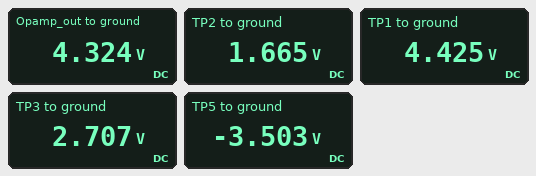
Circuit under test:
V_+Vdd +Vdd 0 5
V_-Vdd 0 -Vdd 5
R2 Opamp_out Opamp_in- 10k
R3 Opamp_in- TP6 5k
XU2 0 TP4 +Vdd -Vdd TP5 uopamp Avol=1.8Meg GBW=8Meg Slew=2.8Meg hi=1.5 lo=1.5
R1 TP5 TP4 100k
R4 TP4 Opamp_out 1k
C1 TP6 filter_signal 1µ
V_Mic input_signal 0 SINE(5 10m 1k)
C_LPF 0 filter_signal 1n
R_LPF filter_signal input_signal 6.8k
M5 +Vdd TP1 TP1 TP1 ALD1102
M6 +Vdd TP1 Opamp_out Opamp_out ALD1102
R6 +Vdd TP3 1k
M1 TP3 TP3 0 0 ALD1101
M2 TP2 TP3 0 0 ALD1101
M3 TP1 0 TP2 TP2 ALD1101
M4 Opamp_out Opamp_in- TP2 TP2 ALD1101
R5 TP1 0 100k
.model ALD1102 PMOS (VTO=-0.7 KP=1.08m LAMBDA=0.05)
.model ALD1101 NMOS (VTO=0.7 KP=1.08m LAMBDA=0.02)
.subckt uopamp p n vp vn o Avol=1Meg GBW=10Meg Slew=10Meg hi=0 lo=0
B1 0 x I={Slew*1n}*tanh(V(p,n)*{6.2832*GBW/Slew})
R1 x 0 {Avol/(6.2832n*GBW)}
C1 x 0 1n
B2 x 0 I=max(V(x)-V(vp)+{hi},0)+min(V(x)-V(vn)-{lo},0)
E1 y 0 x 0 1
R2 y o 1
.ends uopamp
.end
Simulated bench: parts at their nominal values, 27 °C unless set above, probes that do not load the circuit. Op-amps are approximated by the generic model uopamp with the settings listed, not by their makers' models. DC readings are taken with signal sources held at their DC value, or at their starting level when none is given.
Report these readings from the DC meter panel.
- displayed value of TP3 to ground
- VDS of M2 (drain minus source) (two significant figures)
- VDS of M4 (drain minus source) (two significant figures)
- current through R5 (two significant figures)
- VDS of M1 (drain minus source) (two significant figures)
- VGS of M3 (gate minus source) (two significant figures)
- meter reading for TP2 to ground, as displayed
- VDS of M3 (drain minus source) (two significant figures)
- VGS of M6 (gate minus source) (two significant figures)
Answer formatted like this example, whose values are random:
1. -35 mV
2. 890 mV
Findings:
1. 2.707 V
2. 1.7 V
3. 2.7 V
4. 44 µA
5. 2.7 V
6. -1.7 V
7. 1.665 V
8. 2.8 V
9. 100 mV
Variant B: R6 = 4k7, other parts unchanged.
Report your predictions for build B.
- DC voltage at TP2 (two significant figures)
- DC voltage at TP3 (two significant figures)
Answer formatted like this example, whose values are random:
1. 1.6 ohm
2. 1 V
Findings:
1. 2.5 V
2. 1.8 V
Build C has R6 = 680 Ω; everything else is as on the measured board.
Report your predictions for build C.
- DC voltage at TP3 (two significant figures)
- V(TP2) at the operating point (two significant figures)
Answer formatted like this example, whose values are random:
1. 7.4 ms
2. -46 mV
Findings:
1. 3.0 V
2. 1.5 V
